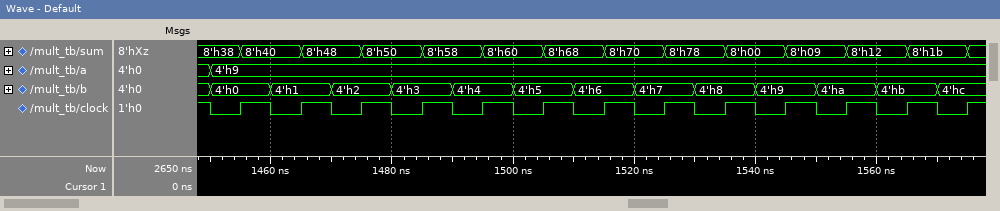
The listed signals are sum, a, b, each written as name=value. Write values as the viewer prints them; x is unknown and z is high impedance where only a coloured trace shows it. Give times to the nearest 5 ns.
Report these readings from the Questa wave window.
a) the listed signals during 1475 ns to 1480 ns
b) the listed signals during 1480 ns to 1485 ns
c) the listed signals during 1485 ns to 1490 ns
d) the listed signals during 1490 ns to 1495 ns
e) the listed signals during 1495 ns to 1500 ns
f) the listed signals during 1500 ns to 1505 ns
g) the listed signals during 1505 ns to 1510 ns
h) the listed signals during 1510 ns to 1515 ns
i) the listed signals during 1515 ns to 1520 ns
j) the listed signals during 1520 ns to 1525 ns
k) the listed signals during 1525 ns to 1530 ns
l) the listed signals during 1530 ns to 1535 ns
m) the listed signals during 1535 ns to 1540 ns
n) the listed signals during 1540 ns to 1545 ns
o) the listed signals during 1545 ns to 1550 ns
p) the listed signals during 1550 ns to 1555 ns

sum=8'h50, a=4'h9, b=4'h2
sum=8'h50, a=4'h9, b=4'h3
sum=8'h58, a=4'h9, b=4'h3
sum=8'h58, a=4'h9, b=4'h4
sum=8'h60, a=4'h9, b=4'h4
sum=8'h60, a=4'h9, b=4'h5
sum=8'h68, a=4'h9, b=4'h5
sum=8'h68, a=4'h9, b=4'h6
sum=8'h70, a=4'h9, b=4'h6
sum=8'h70, a=4'h9, b=4'h7
sum=8'h78, a=4'h9, b=4'h7
sum=8'h78, a=4'h9, b=4'h8
sum=8'h00, a=4'h9, b=4'h8
sum=8'h00, a=4'h9, b=4'h9
sum=8'h09, a=4'h9, b=4'h9
sum=8'h09, a=4'h9, b=4'ha
